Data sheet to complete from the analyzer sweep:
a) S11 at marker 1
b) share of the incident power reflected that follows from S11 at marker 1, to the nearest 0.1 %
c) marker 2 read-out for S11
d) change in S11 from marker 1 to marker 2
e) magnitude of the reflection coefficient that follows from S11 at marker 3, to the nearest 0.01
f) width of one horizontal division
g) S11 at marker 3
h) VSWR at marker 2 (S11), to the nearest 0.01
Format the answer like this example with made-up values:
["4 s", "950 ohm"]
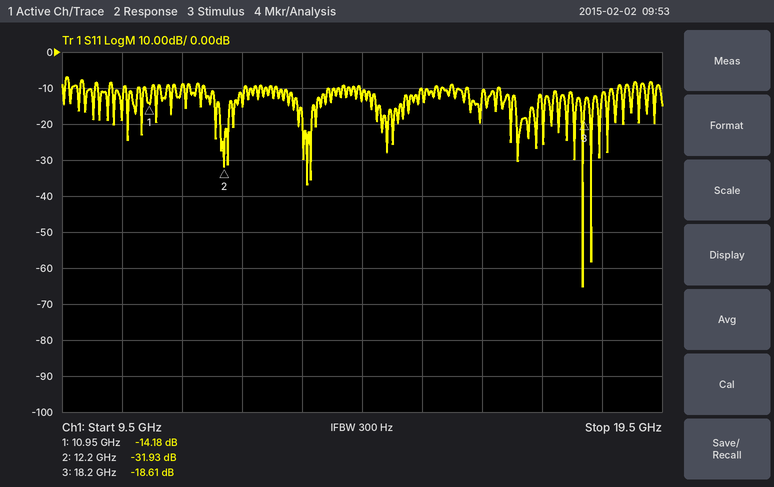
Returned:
["-14.18 dB", "3.8 %", "-31.93 dB", "-17.75 dB", "0.12", "1 GHz", "-18.61 dB", "1.05"]
